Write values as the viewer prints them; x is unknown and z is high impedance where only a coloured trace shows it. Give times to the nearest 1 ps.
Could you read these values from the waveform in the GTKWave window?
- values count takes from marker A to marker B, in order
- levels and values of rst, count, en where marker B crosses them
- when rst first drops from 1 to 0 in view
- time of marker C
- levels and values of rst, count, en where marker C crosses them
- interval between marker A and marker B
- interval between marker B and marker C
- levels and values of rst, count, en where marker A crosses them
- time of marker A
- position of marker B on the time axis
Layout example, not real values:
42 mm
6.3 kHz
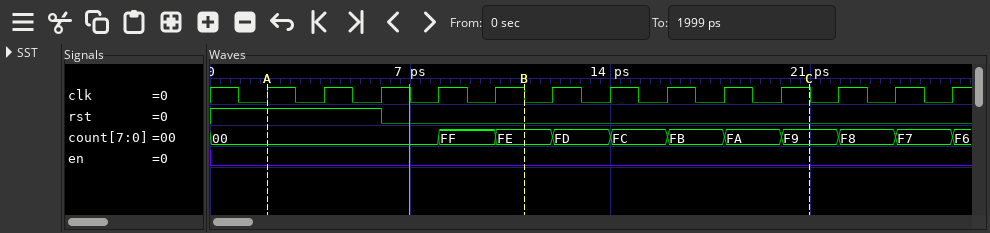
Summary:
00, FF, FE
rst=0, count=FE, en=0
6 ps
21 ps
rst=0, count=F9, en=0
9 ps
10 ps
rst=1, count=00, en=0
2 ps
11 ps
